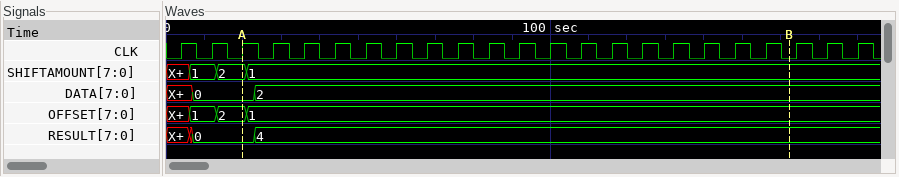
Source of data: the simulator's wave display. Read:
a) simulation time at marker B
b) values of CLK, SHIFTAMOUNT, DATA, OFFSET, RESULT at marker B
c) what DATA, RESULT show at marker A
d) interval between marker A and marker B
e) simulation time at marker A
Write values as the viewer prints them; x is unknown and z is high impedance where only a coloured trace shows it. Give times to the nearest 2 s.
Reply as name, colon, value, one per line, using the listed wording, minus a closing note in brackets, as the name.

simulation time at marker B: 162 s
values of CLK, SHIFTAMOUNT, DATA, OFFSET, RESULT at marker B: CLK=0, SHIFTAMOUNT=1, DATA=2, OFFSET=1, RESULT=4
what DATA, RESULT show at marker A: DATA=0, RESULT=0
interval between marker A and marker B: 142 s
simulation time at marker A: 20 s
